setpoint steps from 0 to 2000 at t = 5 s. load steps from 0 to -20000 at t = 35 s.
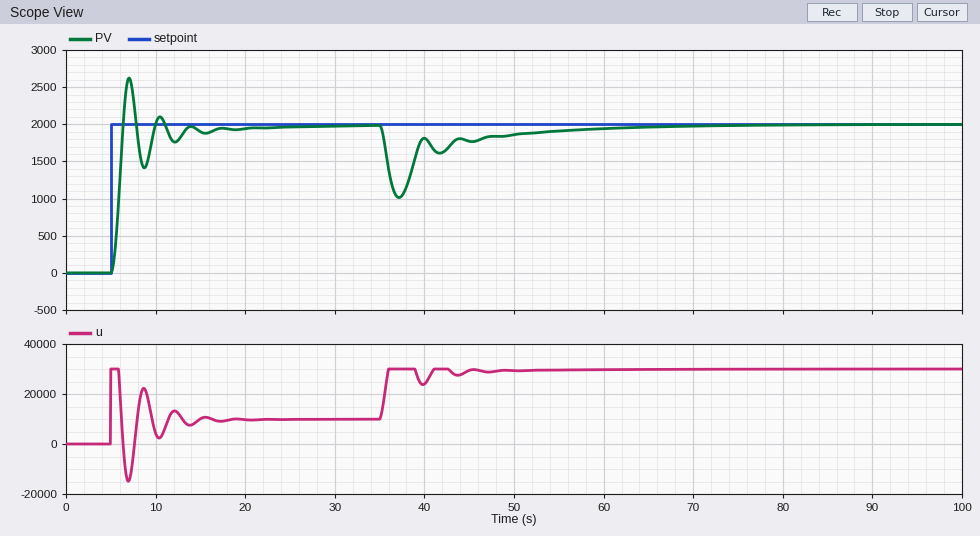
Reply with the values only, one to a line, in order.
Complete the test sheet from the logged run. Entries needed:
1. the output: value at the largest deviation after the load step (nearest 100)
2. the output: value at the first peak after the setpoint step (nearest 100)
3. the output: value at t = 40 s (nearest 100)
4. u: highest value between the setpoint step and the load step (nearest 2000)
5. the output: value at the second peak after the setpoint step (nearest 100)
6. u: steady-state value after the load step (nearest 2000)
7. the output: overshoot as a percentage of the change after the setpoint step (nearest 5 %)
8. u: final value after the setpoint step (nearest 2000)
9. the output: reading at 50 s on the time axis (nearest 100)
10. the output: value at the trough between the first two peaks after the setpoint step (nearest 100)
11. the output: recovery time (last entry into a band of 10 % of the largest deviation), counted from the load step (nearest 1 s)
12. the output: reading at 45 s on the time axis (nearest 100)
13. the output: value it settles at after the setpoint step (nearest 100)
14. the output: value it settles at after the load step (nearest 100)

1000
2600
1800
30000
2100
30000
30 %
10000
1900
1400
19 s
1800
2000
2000
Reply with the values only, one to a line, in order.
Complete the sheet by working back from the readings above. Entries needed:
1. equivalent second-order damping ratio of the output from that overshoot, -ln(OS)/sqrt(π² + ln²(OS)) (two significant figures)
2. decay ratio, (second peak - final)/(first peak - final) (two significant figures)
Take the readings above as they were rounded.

0.36
0.17
